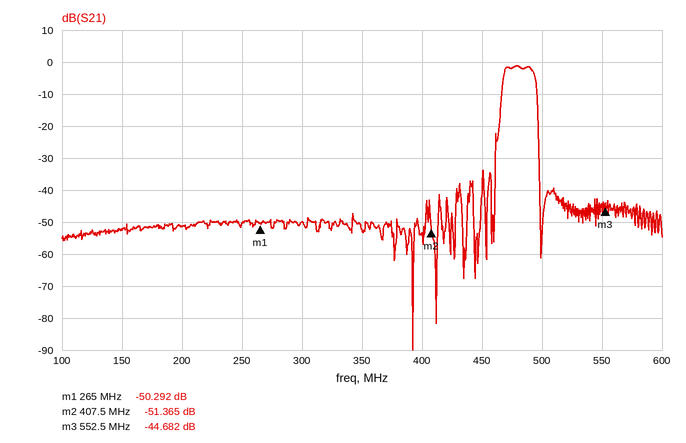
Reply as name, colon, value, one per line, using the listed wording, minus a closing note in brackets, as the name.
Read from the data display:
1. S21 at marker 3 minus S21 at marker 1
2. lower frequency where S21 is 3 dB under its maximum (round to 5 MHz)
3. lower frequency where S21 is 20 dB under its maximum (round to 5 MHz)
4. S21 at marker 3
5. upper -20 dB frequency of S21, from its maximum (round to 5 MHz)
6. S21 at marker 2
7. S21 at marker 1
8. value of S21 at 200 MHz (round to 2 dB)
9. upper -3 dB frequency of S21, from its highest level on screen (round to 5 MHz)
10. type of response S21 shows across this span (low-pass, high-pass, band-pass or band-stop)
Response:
S21 at marker 3 minus S21 at marker 1: 5.610 dB
lower frequency where S21 is 3 dB under its maximum: 470 MHz
lower frequency where S21 is 20 dB under its maximum: 465 MHz
S21 at marker 3: -44.682 dB
upper -20 dB frequency of S21, from its maximum: 495 MHz
S21 at marker 2: -51.365 dB
S21 at marker 1: -50.292 dB
value of S21 at 200 MHz: -52 dB
upper -3 dB frequency of S21, from its highest level on screen: 495 MHz
type of response S21 shows across this span: band-pass
